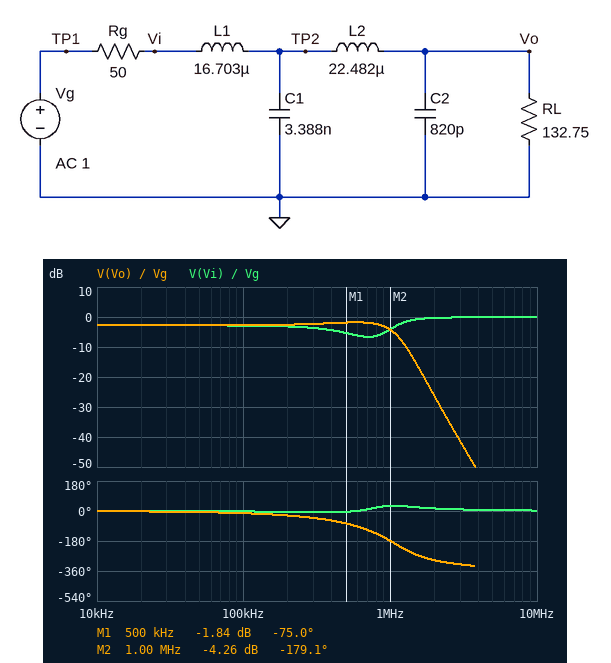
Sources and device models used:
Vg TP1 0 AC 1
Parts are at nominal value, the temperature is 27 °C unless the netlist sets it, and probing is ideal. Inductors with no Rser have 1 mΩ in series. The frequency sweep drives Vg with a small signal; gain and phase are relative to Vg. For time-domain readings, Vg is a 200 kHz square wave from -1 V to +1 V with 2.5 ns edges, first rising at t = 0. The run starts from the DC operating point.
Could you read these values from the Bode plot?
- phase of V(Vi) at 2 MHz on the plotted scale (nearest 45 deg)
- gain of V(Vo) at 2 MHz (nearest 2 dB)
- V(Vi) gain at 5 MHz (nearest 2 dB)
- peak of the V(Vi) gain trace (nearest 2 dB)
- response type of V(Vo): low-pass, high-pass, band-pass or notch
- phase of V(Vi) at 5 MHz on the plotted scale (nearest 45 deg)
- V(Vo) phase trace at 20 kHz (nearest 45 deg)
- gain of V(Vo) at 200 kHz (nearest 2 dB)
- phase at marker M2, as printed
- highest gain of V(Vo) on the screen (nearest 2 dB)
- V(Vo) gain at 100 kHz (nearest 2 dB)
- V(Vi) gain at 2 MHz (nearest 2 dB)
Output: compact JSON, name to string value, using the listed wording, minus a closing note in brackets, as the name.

{"phase of V(Vi) at 2 MHz on the plotted scale": "0 deg", "gain of V(Vo) at 2 MHz": "-26 dB", "V(Vi) gain at 5 MHz": "0 dB", "peak of the V(Vi) gain trace": "0 dB", "response type of V(Vo): low-pass, high-pass, band-pass or notch": "low-pass", "phase of V(Vi) at 5 MHz on the plotted scale": "0 deg", "V(Vo) phase trace at 20 kHz": "0 deg", "gain of V(Vo) at 200 kHz": "-2 dB", "phase at marker M2, as printed": "-179.1 deg", "highest gain of V(Vo) on the screen": "-2 dB", "V(Vo) gain at 100 kHz": "-2 dB", "V(Vi) gain at 2 MHz": "0 dB"}
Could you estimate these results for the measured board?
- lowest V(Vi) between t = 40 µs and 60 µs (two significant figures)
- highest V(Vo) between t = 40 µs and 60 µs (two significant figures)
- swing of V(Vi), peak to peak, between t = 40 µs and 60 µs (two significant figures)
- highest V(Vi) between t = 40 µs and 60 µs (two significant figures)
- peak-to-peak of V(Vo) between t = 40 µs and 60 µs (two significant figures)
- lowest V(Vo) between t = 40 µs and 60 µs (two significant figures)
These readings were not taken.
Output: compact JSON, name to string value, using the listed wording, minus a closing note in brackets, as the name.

{"lowest V(Vi) between t = 40 µs and 60 µs": "-1.3 V", "highest V(Vo) between t = 40 µs and 60 µs": "1.0 V", "swing of V(Vi), peak to peak, between t = 40 µs and 60 µs": "2.5 V", "highest V(Vi) between t = 40 µs and 60 µs": "1.3 V", "peak-to-peak of V(Vo) between t = 40 µs and 60 µs": "2.0 V", "lowest V(Vo) between t = 40 µs and 60 µs": "-1.0 V"}
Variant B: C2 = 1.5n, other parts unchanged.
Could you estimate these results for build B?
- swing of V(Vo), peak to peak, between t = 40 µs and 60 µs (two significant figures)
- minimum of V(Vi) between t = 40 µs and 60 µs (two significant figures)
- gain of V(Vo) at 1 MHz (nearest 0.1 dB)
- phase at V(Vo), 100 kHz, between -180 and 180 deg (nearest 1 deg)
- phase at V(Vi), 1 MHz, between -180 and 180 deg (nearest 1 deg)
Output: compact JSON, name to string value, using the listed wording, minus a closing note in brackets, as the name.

{"swing of V(Vo), peak to peak, between t = 40 µs and 60 µs": "2.1 V", "minimum of V(Vi) between t = 40 µs and 60 µs": "-1.3 V", "gain of V(Vo) at 1 MHz": "-2.9 dB", "phase at V(Vo), 100 kHz, between -180 and 180 deg": "-14 deg", "phase at V(Vi), 1 MHz, between -180 and 180 deg": "25 deg"}
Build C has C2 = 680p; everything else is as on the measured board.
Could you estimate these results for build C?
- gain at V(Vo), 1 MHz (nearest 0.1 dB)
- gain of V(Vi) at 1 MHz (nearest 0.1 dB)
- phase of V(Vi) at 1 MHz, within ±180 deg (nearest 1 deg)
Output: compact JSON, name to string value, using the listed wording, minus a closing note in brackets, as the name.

{"gain at V(Vo), 1 MHz": "-4.6 dB", "gain of V(Vi) at 1 MHz": "-4.0 dB", "phase of V(Vi) at 1 MHz, within ±180 deg": "33 deg"}
